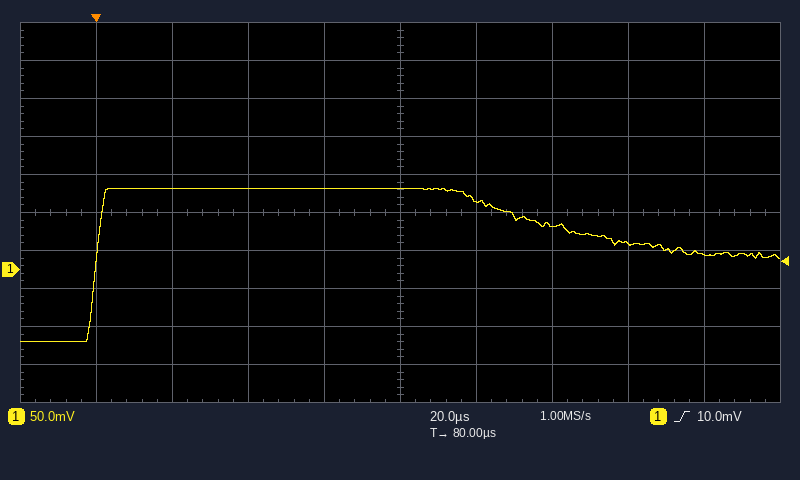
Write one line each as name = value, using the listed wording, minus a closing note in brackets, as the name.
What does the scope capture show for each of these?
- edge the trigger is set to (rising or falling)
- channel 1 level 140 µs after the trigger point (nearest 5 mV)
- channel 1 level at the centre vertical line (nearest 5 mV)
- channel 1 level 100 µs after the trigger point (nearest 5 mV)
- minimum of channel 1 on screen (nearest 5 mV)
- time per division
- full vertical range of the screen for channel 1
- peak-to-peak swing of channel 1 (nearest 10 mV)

edge the trigger is set to = rising
channel 1 level 140 µs after the trigger point = 35 mV
channel 1 level at the centre vertical line = 105 mV
channel 1 level 100 µs after the trigger point = 90 mV
minimum of channel 1 on screen = -95 mV
time per division = 20 µs
full vertical range of the screen for channel 1 = 500 mV
peak-to-peak swing of channel 1 = 200 mV
